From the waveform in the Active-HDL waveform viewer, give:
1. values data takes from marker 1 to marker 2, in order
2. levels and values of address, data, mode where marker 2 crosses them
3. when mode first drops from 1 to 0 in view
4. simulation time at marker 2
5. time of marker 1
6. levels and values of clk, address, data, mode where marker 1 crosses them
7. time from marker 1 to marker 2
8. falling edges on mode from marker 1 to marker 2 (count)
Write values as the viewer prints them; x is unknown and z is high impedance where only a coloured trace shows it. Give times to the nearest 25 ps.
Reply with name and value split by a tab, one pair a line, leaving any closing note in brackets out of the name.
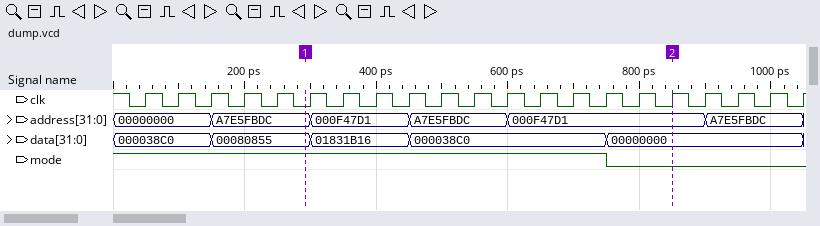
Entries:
values data takes from marker 1 to marker 2, in order	00080855, 01831B16, 000038C0, 00000000
levels and values of address, data, mode where marker 2 crosses them	address=000F47D1, data=00000000, mode=0
when mode first drops from 1 to 0 in view	750 ps
simulation time at marker 2	850 ps
time of marker 1	300 ps
levels and values of clk, address, data, mode where marker 1 crosses them	clk=0, address=A7E5FBDC, data=00080855, mode=1
time from marker 1 to marker 2	550 ps
falling edges on mode from marker 1 to marker 2	1
